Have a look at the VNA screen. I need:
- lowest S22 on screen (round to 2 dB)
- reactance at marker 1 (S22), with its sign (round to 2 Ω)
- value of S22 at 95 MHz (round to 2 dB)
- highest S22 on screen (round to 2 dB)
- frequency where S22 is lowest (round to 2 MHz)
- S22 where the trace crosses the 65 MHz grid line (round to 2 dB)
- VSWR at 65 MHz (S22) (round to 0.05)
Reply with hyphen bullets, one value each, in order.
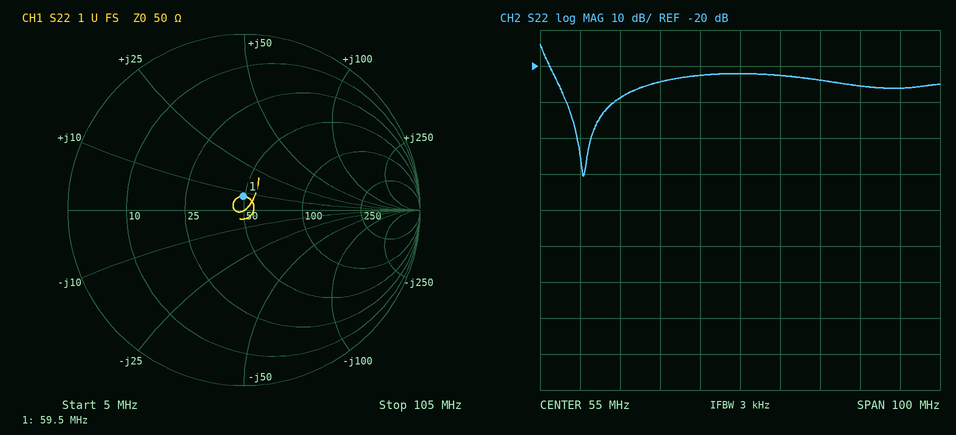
- -50 dB
- +8 Ω
- -26 dB
- -14 dB
- 16 MHz
- -22 dB
- 1.15
